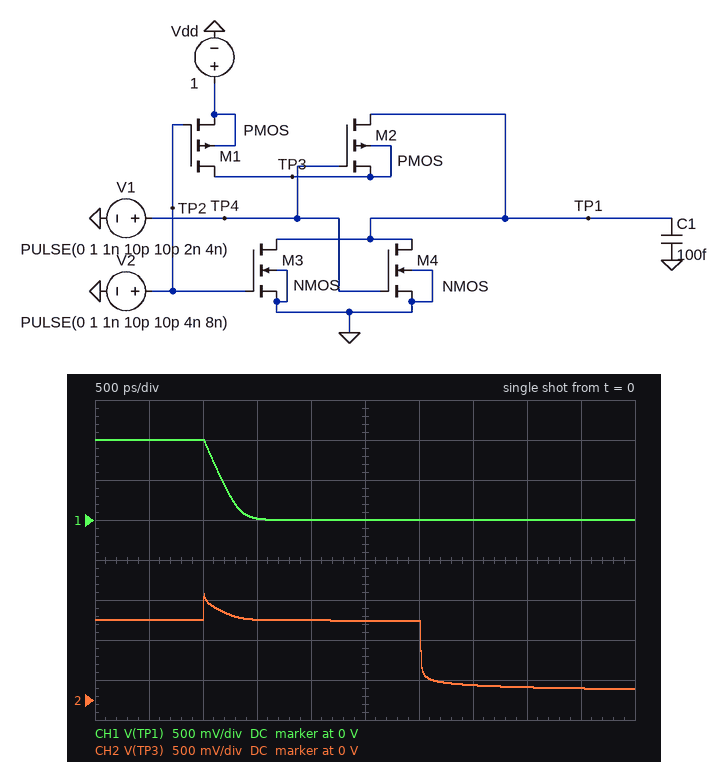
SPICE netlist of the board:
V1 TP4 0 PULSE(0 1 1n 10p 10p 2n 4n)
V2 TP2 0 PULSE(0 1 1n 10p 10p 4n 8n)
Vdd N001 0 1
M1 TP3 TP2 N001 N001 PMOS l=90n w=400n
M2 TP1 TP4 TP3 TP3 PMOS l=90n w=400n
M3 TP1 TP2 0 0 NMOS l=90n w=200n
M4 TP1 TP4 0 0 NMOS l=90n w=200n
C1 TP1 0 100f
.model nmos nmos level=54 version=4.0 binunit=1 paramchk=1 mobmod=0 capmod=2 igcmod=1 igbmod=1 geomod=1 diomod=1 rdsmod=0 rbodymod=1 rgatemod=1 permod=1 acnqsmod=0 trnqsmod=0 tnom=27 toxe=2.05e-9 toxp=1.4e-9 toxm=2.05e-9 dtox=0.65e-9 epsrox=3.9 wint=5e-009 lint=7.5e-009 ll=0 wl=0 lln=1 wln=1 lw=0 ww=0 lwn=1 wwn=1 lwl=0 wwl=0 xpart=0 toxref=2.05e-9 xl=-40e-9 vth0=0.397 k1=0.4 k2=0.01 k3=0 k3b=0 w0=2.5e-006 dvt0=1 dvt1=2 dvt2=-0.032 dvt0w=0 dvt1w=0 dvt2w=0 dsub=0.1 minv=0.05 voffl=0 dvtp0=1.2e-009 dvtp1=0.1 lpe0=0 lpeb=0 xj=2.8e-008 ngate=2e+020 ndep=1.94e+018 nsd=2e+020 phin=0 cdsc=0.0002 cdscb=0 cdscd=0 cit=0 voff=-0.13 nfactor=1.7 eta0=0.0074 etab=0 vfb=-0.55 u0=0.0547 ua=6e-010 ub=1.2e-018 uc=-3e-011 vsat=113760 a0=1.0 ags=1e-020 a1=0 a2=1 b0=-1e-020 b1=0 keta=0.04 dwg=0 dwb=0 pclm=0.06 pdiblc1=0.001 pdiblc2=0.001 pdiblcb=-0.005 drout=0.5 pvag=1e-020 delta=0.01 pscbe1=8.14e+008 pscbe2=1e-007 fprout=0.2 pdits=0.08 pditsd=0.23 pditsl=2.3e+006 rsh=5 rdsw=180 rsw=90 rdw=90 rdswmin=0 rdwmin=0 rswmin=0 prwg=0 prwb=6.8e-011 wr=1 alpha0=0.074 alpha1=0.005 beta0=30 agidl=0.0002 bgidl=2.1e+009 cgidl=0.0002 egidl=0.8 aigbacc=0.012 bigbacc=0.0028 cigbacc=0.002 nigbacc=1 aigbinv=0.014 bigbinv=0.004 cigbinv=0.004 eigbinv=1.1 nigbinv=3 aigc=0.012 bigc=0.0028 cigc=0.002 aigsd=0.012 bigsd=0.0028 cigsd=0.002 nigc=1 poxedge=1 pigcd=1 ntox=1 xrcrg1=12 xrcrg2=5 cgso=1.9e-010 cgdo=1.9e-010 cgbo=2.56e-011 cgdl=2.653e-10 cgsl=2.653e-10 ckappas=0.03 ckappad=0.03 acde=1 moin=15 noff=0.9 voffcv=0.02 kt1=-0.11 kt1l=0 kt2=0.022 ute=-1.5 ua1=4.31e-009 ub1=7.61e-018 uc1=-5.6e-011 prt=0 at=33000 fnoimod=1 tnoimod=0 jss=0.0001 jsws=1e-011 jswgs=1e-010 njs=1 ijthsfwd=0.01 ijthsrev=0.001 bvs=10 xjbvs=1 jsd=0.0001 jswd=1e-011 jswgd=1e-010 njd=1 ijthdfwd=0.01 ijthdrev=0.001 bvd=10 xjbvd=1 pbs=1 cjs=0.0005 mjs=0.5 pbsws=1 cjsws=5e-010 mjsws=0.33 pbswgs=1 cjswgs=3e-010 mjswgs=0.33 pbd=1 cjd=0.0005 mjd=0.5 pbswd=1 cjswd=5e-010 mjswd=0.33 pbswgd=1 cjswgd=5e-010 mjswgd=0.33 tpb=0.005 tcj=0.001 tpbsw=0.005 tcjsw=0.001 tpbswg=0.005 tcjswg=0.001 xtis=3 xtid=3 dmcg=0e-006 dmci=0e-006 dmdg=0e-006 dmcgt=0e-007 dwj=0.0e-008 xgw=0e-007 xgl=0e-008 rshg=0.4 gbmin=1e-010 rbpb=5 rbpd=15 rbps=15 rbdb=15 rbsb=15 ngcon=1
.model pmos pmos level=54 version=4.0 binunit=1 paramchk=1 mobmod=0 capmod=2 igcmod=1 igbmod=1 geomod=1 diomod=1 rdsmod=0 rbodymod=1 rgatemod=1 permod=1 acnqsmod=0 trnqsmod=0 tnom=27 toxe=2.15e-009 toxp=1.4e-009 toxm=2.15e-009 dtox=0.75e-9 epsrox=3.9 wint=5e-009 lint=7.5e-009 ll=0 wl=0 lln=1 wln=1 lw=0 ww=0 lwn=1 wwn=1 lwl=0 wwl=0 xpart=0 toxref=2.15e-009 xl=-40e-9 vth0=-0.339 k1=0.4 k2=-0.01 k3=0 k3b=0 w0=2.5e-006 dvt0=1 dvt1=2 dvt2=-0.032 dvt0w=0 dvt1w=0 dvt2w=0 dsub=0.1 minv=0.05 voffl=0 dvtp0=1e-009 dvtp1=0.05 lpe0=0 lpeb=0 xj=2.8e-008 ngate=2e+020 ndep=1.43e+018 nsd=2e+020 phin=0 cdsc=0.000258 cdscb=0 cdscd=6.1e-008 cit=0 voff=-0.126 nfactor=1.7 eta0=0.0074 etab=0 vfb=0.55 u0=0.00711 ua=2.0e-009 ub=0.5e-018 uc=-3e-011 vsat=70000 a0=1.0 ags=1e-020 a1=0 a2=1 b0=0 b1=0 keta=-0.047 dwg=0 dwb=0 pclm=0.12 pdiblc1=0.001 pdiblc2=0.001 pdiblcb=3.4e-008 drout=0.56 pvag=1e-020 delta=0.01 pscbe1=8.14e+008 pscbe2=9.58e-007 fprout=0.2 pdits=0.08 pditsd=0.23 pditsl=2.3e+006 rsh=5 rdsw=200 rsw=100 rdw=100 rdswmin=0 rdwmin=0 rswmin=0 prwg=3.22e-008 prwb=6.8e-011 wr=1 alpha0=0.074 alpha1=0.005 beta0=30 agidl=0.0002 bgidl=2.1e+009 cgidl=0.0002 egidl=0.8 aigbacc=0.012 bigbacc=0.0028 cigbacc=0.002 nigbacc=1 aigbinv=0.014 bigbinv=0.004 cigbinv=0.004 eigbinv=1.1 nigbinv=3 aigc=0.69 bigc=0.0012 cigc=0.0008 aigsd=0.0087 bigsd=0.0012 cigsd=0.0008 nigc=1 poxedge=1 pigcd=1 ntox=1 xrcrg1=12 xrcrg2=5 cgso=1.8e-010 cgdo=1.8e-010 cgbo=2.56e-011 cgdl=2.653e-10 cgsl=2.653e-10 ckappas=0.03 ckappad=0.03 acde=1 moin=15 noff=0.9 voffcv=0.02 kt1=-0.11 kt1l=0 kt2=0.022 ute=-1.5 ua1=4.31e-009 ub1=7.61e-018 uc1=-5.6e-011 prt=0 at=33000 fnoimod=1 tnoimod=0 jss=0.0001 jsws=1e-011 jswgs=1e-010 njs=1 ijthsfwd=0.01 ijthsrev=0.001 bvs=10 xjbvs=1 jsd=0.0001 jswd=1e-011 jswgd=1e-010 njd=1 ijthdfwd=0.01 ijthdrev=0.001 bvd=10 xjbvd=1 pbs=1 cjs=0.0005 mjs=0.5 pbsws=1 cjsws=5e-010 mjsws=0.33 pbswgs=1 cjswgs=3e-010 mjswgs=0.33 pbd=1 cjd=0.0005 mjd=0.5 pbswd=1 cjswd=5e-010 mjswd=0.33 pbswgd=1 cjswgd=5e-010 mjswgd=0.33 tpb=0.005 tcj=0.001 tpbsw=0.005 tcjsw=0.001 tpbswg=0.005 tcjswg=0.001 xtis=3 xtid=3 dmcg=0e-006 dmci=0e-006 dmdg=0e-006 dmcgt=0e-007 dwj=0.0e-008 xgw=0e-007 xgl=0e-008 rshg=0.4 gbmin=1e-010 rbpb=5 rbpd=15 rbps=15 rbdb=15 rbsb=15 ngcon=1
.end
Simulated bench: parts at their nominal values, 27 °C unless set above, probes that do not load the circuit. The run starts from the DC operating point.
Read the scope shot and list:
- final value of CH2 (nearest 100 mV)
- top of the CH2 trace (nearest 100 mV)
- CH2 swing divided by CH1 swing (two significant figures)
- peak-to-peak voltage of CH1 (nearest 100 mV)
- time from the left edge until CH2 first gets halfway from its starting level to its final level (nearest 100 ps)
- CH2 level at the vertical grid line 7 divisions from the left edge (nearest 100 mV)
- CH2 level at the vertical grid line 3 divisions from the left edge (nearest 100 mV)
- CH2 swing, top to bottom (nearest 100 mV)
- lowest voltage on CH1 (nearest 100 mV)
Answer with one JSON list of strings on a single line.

["100 mV", "1.3 V", "1.2", "1.0 V", "3.0 ns", "200 mV", "1.0 V", "1.2 V", "0 V"]
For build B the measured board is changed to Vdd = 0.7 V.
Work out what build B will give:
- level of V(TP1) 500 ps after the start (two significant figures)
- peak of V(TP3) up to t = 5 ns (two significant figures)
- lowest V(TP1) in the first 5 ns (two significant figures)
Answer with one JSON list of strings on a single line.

["700 mV", "1.2 V", "-2.8 mV"]
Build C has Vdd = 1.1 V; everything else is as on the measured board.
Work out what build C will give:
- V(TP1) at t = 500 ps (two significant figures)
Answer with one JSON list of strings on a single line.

["1.1 V"]
